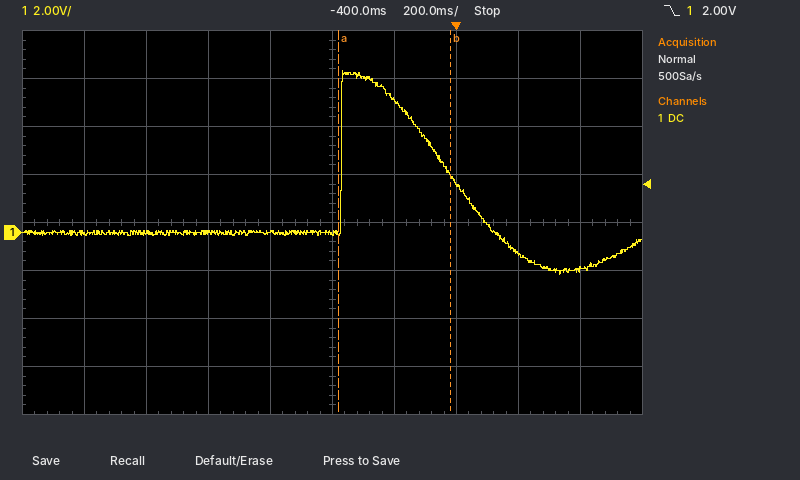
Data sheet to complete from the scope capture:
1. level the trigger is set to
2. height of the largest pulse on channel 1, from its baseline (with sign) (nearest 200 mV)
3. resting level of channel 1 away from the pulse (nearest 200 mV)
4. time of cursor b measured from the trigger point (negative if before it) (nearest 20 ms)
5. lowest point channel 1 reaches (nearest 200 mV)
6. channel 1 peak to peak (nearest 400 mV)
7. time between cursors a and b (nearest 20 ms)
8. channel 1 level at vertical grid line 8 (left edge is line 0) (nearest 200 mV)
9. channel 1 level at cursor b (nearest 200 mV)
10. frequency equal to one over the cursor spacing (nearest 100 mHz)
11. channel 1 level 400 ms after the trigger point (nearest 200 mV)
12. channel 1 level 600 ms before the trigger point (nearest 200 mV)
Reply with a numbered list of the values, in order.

1. 2.00 V
2. +6.8 V
3. 0.0 V
4. -20 ms
5. -1.8 V
6. 8.4 V
7. 360 ms
8. -800 mV
9. 2.4 V
10. 2.8 Hz
11. -1.6 V
12. 0.0 V
